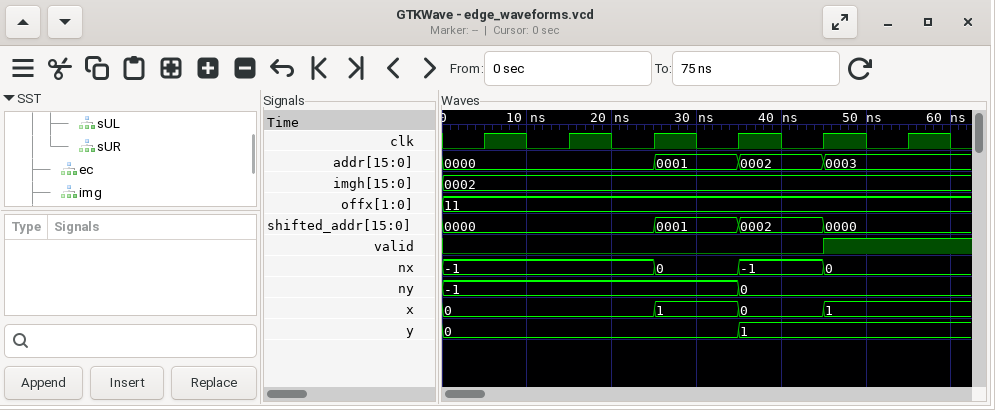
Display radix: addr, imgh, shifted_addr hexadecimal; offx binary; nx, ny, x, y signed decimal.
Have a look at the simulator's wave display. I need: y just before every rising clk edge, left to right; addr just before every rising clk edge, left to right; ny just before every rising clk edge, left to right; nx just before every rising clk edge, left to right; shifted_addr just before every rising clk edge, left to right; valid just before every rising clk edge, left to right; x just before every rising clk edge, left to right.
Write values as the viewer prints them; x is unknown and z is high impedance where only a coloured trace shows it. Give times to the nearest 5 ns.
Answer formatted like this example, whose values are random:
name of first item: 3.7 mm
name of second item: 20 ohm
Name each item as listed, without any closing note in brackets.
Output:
y just before every rising clk edge, left to right: 0, 0, 0, 0, 1, 1
addr just before every rising clk edge, left to right: 0000, 0000, 0000, 0001, 0002, 0003
ny just before every rising clk edge, left to right: -1, -1, -1, -1, 0, 0
nx just before every rising clk edge, left to right: -1, -1, -1, 0, -1, 0
shifted_addr just before every rising clk edge, left to right: 0000, 0000, 0000, 0001, 0002, 0000
valid just before every rising clk edge, left to right: 0 0 0 0 0 1
x just before every rising clk edge, left to right: 0, 0, 0, 1, 0, 1
